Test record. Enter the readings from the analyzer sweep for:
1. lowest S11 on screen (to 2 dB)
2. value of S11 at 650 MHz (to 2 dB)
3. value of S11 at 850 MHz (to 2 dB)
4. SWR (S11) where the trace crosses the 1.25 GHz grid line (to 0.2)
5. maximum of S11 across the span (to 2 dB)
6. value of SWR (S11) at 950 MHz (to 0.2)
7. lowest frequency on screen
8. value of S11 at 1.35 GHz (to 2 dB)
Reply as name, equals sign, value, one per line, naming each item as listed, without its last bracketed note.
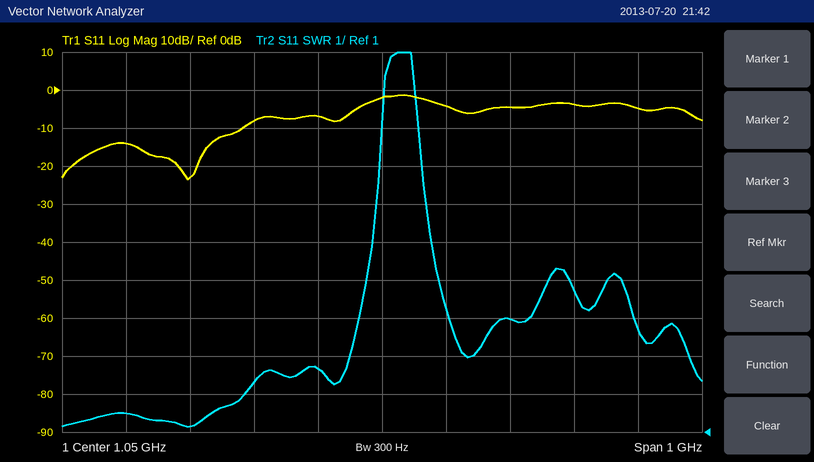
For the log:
lowest S11 on screen = -24 dB
value of S11 at 650 MHz = -14 dB
value of S11 at 850 MHz = -8 dB
SWR (S11) where the trace crosses the 1.25 GHz grid line = 4.0
maximum of S11 across the span = -2 dB
value of SWR (S11) at 950 MHz = 2.6
lowest frequency on screen = 550 MHz
value of S11 at 1.35 GHz = -4 dB
